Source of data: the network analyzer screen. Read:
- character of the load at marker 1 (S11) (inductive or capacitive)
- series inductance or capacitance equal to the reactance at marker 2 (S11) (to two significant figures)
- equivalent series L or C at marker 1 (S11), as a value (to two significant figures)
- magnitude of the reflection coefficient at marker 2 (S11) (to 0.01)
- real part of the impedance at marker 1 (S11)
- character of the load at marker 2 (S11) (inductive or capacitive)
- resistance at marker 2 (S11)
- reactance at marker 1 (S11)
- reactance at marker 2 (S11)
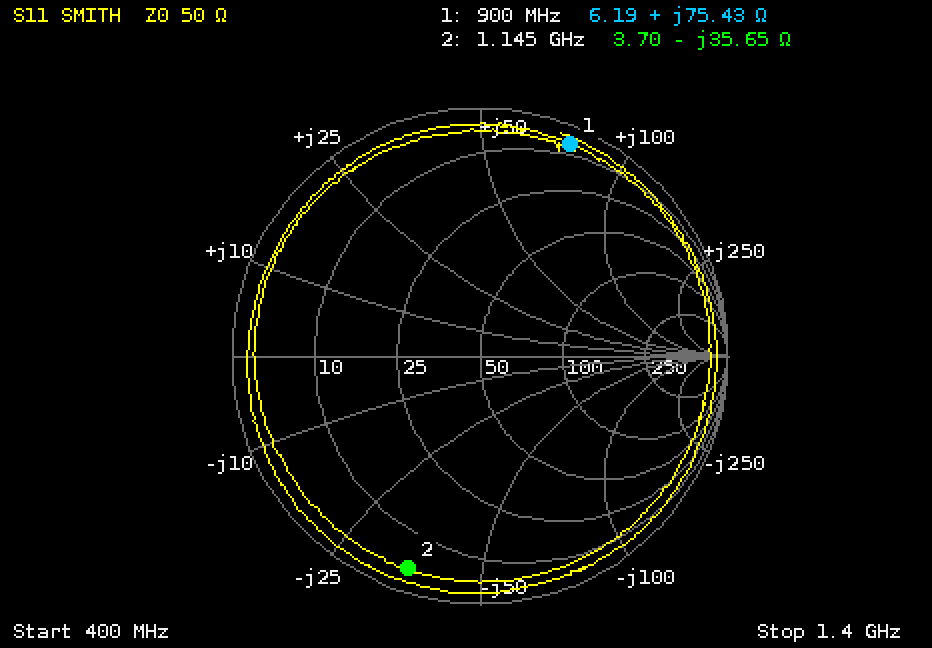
inductive
3.9 pF
13 nH
0.91
6.19 Ω
capacitive
3.70 Ω
+75.43 Ω
-35.65 Ω
